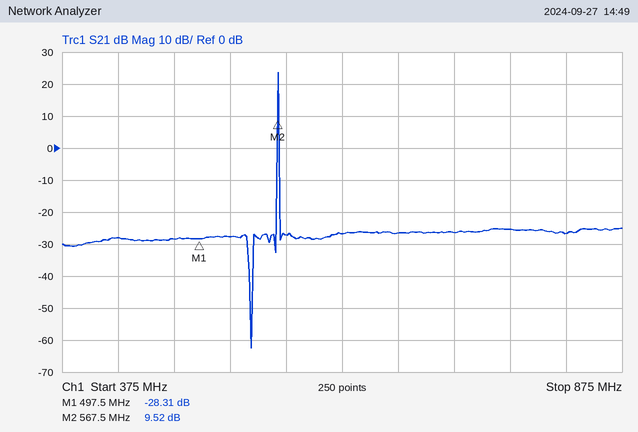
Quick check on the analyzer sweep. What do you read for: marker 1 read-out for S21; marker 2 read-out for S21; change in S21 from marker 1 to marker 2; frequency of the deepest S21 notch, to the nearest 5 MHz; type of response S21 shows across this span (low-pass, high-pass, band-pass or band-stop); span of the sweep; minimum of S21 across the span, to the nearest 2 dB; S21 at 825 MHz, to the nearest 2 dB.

-28.31 dB
9.52 dB
37.83 dB
545 MHz
band-pass
500 MHz
-62 dB
-26 dB
